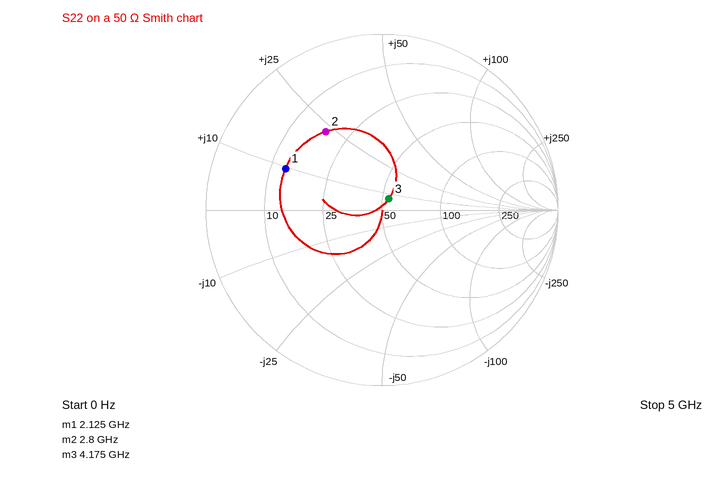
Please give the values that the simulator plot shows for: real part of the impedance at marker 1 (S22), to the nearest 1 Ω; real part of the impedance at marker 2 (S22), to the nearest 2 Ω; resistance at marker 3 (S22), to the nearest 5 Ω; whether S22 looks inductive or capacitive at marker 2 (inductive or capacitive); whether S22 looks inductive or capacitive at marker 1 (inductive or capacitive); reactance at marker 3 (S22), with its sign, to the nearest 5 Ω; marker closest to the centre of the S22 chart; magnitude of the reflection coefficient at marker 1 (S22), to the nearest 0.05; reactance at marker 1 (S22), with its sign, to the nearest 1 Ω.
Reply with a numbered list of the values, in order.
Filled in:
1. 13 Ω
2. 18 Ω
3. 55 Ω
4. inductive
5. inductive
6. +5 Ω
7. marker 3
8. 0.60
9. +10 Ω
